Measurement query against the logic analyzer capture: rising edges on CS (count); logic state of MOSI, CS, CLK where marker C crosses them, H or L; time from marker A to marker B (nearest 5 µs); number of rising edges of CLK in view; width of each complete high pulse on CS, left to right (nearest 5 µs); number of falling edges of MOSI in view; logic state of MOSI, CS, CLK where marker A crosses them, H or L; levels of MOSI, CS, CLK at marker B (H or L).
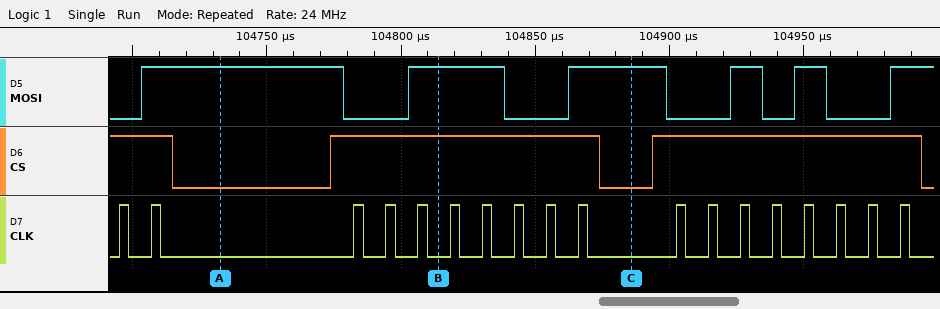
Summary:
2
MOSI=H, CS=L, CLK=L
80 µs
18
100 µs, 100 µs
5
MOSI=H, CS=L, CLK=L
MOSI=H, CS=H, CLK=L
